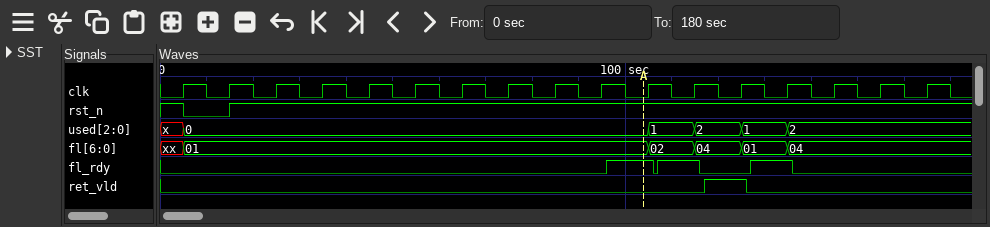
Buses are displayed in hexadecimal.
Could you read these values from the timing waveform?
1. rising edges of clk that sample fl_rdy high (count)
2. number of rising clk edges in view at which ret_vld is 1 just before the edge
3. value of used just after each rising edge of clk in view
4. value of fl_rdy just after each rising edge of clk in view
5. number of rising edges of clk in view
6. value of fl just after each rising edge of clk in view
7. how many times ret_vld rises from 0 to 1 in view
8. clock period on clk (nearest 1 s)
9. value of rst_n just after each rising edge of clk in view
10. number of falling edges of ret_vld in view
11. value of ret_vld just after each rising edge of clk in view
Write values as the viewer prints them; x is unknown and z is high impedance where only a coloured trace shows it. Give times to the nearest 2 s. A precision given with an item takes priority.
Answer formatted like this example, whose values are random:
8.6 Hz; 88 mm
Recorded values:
3; 1; 0, 0, 0, 0, 0, 0, 0, 0, 0, 0, 1, 2, 1, 2, 2, 2, 2; 0 0 0 0 0 0 0 0 0 0 1 1 0 1 0 0 0; 17; 01, 01, 01, 01, 01, 01, 01, 01, 01, 01, 02, 04, 01, 04, 04, 04, 04; 1; 10 s; 0 1 1 1 1 1 1 1 1 1 1 1 1 1 1 1 1; 1; 0 0 0 0 0 0 0 0 0 0 0 0 1 0 0 0 0
